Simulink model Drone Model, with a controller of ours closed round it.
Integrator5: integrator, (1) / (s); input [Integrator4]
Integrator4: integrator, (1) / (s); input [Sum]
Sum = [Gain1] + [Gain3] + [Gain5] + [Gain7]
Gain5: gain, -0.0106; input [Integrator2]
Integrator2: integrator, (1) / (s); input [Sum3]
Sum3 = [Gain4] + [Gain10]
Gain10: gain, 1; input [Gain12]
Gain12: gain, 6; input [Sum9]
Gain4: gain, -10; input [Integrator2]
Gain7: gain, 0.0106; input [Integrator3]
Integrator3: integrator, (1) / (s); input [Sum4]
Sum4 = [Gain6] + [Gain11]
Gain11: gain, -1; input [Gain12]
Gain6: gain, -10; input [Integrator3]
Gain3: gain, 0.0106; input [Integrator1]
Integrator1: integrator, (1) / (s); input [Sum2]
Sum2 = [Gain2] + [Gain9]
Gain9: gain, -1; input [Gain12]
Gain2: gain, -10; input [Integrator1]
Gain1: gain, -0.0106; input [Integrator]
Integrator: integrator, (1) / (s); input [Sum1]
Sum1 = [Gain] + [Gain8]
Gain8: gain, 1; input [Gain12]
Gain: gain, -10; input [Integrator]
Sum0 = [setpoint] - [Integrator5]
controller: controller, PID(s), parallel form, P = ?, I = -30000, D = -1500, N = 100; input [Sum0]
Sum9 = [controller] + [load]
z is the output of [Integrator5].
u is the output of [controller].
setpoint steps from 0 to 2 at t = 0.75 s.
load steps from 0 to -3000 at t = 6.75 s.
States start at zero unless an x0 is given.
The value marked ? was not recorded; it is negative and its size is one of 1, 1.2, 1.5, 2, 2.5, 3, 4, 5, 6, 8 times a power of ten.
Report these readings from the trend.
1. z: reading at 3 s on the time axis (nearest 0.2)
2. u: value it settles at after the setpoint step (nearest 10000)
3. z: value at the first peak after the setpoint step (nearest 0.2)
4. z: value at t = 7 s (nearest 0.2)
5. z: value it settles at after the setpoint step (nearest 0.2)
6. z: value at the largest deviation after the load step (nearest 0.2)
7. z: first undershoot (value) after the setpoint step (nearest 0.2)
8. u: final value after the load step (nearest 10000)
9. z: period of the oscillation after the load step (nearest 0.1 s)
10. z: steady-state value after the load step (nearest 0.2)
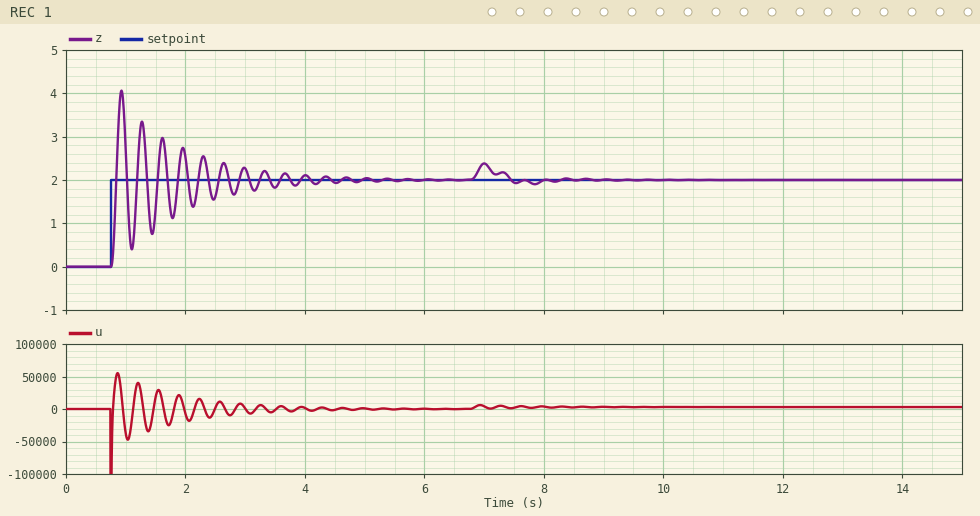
2.2
0
4.0
2.4
2.0
2.4
0.4
0
0.3 s
2.0
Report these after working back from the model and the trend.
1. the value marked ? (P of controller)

-6000
